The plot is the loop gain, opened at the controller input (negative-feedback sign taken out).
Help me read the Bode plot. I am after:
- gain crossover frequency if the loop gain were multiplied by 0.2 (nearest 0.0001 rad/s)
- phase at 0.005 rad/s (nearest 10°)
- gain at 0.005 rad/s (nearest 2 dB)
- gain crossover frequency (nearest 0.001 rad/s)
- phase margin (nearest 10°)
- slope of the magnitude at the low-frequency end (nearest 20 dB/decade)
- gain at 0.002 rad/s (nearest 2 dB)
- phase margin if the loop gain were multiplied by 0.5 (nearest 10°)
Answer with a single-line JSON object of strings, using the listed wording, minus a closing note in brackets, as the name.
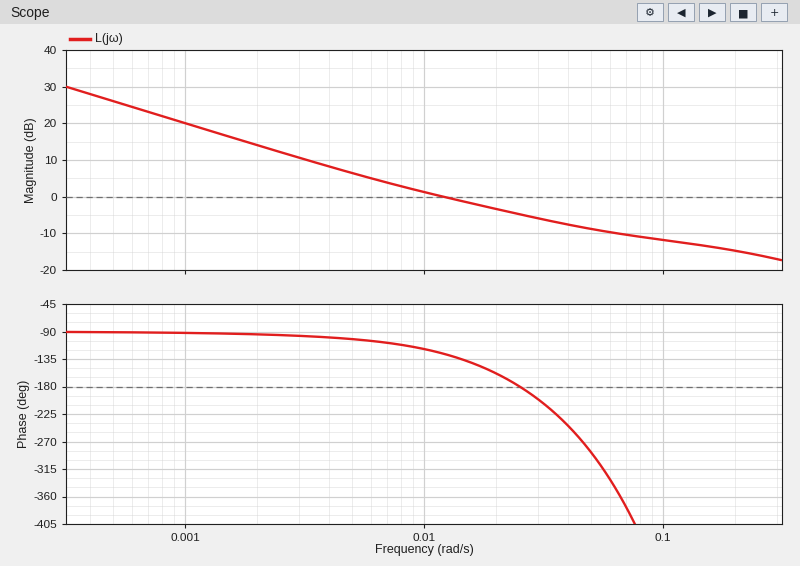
{"gain crossover frequency if the loop gain were multiplied by 0.2": "0.0020 rad/s", "phase at 0.005 rad/s": "-100°", "gain at 0.005 rad/s": "6 dB", "gain crossover frequency": "0.012 rad/s", "phase margin": "50°", "slope of the magnitude at the low-frequency end": "-20 dB/decade", "gain at 0.002 rad/s": "14 dB", "phase margin if the loop gain were multiplied by 0.5": "80°"}
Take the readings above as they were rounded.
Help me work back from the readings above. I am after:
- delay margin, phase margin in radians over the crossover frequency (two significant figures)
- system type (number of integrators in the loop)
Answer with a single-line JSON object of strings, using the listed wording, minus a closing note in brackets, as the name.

{"delay margin, phase margin in radians over the crossover frequency": "73 s", "system type": "1"}
